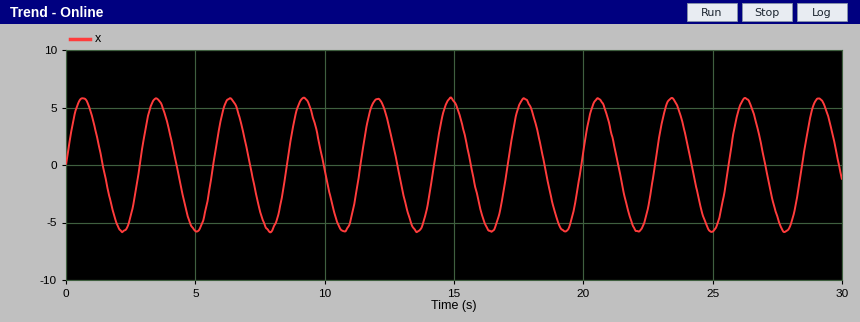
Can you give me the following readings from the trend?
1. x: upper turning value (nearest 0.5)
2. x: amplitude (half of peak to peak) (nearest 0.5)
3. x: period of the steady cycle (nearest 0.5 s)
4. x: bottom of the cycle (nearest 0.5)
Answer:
6.0
6.0
3.0 s
-6.0
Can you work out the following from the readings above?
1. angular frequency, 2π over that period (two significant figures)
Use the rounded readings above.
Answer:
2.1 rad/s
